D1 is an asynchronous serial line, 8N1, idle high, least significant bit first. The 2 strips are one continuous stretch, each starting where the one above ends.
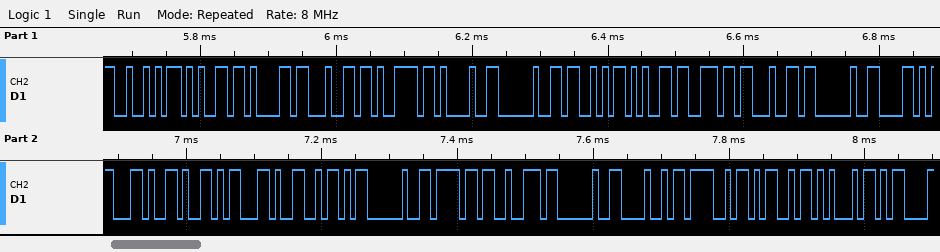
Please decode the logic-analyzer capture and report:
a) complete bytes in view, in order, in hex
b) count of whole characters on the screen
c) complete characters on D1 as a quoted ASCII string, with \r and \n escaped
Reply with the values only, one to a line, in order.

52 65 61 64 79 21 20 53 65 6E 64 20 58 2C 59 2C 5A 20 6F 72 20 48 4F 4D 45 0D
26
"Ready! Send X,Y,Z or HOME\r"
